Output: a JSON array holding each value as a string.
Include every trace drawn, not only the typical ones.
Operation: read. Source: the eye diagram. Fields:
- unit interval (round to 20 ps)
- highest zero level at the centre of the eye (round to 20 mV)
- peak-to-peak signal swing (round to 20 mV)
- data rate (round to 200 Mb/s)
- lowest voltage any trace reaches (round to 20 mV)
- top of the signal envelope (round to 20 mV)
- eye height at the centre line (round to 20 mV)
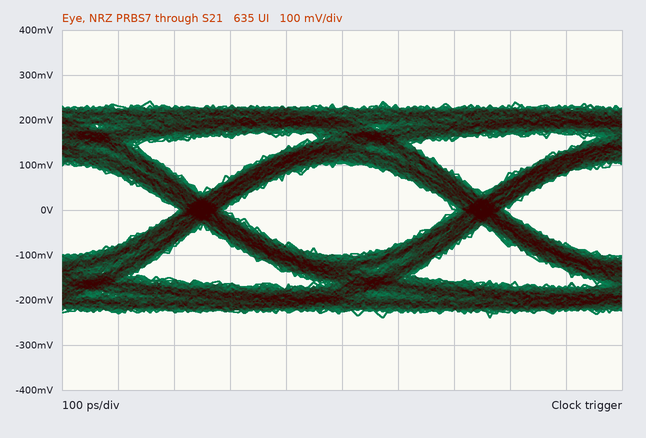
["500 ps", "-100 mV", "480 mV", "2.0 Gb/s", "-240 mV", "240 mV", "200 mV"]
